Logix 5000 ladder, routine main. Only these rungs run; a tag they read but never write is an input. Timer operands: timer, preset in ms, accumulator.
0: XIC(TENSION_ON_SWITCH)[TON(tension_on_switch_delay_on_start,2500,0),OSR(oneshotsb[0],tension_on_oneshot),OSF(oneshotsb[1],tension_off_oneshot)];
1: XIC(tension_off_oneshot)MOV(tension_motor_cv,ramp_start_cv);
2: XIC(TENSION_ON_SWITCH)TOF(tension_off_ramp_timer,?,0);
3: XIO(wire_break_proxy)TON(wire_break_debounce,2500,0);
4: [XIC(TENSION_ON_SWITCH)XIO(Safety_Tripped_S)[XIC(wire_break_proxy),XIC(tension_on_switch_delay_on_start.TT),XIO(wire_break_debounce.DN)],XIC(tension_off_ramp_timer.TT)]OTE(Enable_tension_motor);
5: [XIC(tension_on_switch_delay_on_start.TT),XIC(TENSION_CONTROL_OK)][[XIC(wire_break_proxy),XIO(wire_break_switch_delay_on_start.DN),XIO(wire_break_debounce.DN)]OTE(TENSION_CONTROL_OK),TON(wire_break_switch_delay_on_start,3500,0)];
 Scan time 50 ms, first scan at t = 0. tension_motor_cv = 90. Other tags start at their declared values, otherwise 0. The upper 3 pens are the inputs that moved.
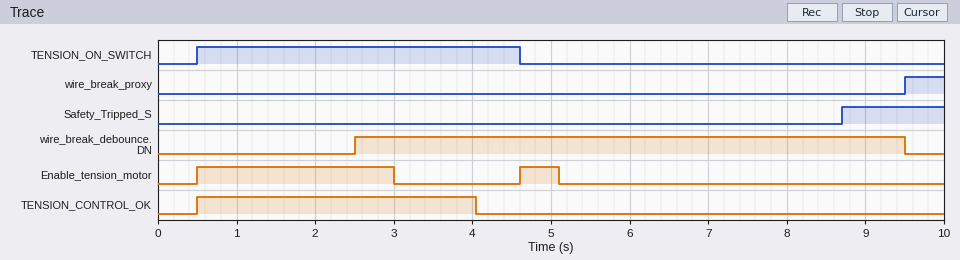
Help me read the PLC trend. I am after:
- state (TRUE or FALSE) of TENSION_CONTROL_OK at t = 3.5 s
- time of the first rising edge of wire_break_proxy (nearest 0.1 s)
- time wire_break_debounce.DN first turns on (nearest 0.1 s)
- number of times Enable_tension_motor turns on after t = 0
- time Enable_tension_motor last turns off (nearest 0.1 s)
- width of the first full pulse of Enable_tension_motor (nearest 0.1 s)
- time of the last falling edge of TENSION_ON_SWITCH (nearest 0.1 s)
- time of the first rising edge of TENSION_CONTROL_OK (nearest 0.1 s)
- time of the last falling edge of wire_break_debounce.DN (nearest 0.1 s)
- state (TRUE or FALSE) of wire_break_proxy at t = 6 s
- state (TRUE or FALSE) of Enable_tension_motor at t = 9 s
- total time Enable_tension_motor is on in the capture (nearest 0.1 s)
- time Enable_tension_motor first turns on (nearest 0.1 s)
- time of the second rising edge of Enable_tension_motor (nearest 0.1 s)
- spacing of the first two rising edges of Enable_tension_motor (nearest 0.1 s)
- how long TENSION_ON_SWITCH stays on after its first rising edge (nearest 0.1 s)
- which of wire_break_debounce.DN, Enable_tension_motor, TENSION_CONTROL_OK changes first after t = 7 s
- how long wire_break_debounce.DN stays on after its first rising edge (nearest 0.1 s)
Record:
TRUE
9.5 s
2.5 s
2
5.1 s
2.5 s
4.6 s
0.5 s
9.5 s
FALSE
FALSE
3.0 s
0.5 s
4.6 s
4.1 s
4.1 s
wire_break_debounce.DN
7.0 s
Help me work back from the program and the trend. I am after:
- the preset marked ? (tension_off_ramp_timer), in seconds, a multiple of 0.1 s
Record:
0.5 s
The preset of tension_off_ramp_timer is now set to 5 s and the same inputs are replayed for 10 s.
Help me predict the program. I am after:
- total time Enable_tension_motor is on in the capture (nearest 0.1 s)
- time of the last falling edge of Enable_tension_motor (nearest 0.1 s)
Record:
7.5 s
9.6 s
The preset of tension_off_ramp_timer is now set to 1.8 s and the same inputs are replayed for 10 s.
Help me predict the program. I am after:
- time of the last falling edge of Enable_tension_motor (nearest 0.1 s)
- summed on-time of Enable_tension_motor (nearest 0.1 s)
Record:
6.4 s
4.3 s
